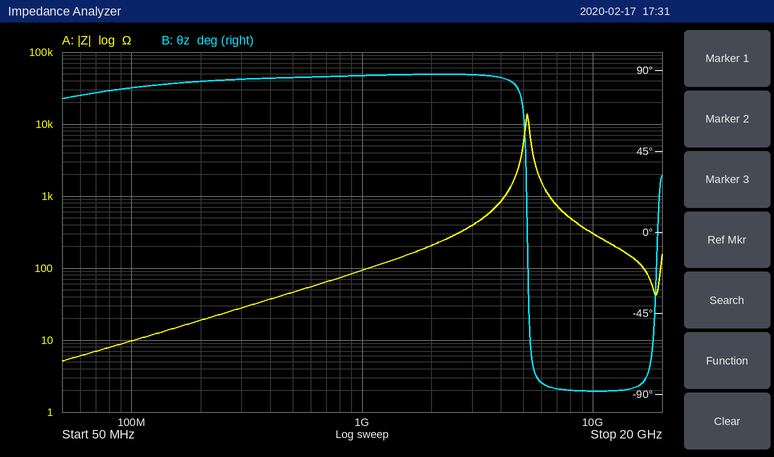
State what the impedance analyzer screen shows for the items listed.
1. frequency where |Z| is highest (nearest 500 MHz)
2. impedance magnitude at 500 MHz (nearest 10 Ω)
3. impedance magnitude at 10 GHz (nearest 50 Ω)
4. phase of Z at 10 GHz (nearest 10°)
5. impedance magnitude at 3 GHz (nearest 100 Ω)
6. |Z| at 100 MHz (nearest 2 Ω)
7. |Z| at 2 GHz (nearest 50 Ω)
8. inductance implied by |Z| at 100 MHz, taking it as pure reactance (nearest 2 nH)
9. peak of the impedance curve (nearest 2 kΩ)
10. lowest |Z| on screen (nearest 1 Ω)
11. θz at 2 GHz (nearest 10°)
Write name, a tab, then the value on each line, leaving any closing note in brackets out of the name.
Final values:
frequency where |Z| is highest	5.0 GHz
impedance magnitude at 500 MHz	50 Ω
impedance magnitude at 10 GHz	300 Ω
phase of Z at 10 GHz	-90°
impedance magnitude at 3 GHz	400 Ω
|Z| at 100 MHz	10 Ω
|Z| at 2 GHz	200 Ω
inductance implied by |Z| at 100 MHz, taking it as pure reactance	16 nH
peak of the impedance curve	14 kΩ
lowest |Z| on screen	5 Ω
θz at 2 GHz	90°
